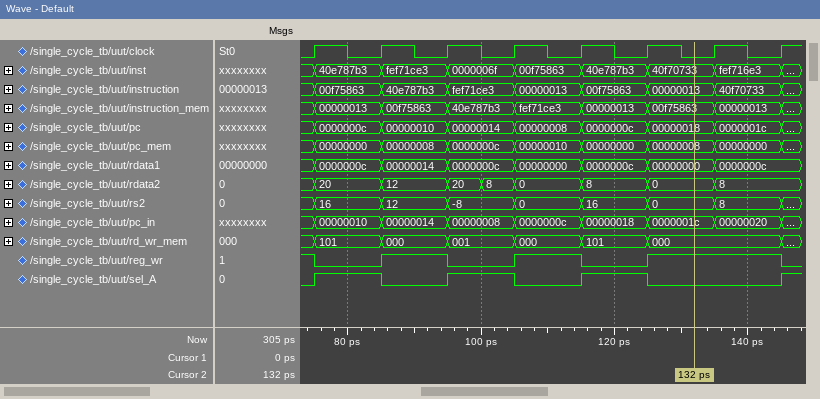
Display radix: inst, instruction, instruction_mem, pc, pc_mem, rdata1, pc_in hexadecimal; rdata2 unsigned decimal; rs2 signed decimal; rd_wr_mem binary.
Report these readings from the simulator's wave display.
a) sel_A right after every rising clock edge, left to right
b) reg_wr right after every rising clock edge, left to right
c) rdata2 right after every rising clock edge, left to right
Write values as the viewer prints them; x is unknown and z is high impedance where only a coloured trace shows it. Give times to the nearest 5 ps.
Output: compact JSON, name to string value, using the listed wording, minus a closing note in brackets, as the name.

{"sel_A right after every rising clock edge, left to right": "1 0 1 0 1 0 0 1", "reg_wr right after every rising clock edge, left to right": "0 1 0 1 0 1 1 0", "rdata2 right after every rising clock edge, left to right": "20, 12, 20, 0, 8, 0, 8, 8"}
